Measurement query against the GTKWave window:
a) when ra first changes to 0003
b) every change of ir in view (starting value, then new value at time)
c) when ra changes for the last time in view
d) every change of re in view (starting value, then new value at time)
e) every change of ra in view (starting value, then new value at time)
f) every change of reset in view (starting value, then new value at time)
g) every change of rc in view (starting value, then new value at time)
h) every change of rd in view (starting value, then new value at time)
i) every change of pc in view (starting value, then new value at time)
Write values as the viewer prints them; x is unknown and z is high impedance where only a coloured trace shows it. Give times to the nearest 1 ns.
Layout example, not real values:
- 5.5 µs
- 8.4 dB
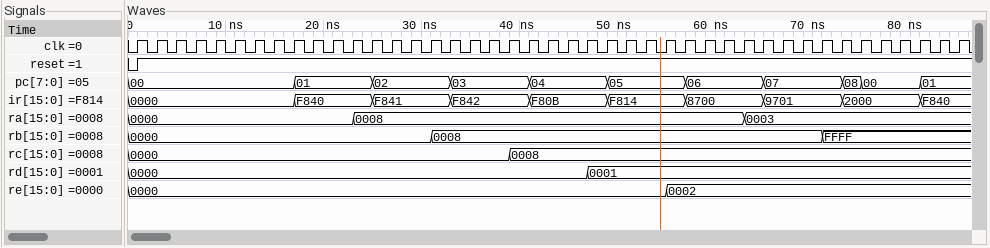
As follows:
- 63 ns
- 0000, F840 at 17 ns, F841 at 25 ns, F842 at 33 ns, F80B at 41 ns, F814 at 49 ns, 8700 at 57 ns, 9701 at 65 ns, 2000 at 73 ns, F840 at 81 ns
- 63 ns
- 0000, 0002 at 55 ns
- 0000, 0008 at 23 ns, 0003 at 63 ns
- 0, 1 at 1 ns
- 0000, 0008 at 39 ns
- 0000, 0001 at 47 ns
- 00, 01 at 17 ns, 02 at 25 ns, 03 at 33 ns, 04 at 41 ns, 05 at 49 ns, 06 at 57 ns, 07 at 65 ns, 08 at 73 ns, 00 at 75 ns, 01 at 81 ns
